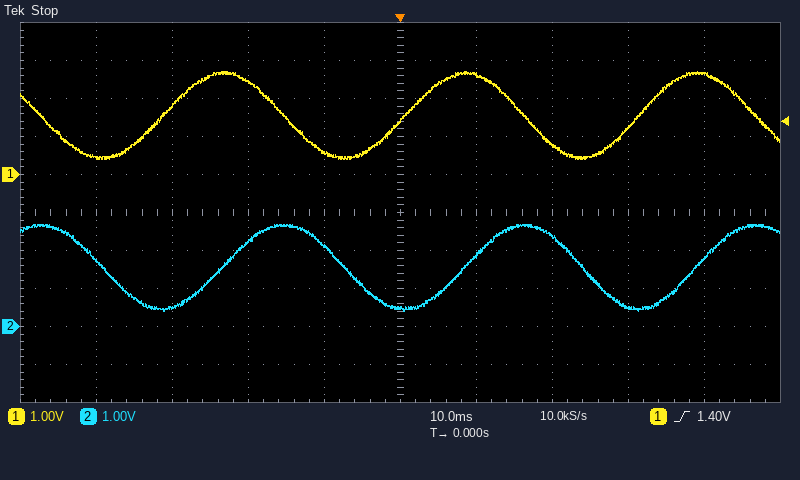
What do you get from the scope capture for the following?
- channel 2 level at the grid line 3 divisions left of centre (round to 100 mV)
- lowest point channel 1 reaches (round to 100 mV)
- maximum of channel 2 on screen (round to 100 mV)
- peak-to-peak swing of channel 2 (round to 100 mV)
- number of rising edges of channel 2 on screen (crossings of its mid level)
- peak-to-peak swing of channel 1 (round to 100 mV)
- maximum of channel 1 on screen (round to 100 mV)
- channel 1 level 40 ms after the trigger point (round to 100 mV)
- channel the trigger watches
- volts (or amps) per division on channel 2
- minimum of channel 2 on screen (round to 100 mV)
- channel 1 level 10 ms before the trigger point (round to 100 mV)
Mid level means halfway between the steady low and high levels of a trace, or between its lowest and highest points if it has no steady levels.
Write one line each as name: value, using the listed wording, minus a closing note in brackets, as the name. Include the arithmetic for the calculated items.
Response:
channel 2 level at the grid line 3 divisions left of centre: 500 mV
lowest point channel 1 reaches: 400 mV
maximum of channel 2 on screen: 2.7 V
peak-to-peak swing of channel 2: 2.7 V − (400 mV) = 2.3 V
number of rising edges of channel 2 on screen: 3
peak-to-peak swing of channel 1: 2.7 V − (400 mV) = 2.3 V
maximum of channel 1 on screen: 2.7 V
channel 1 level 40 ms after the trigger point: 2.6 V
channel the trigger watches: channel 1
volts (or amps) per division on channel 2: 1 V
minimum of channel 2 on screen: 400 mV
channel 1 level 10 ms before the trigger point: 600 mV
